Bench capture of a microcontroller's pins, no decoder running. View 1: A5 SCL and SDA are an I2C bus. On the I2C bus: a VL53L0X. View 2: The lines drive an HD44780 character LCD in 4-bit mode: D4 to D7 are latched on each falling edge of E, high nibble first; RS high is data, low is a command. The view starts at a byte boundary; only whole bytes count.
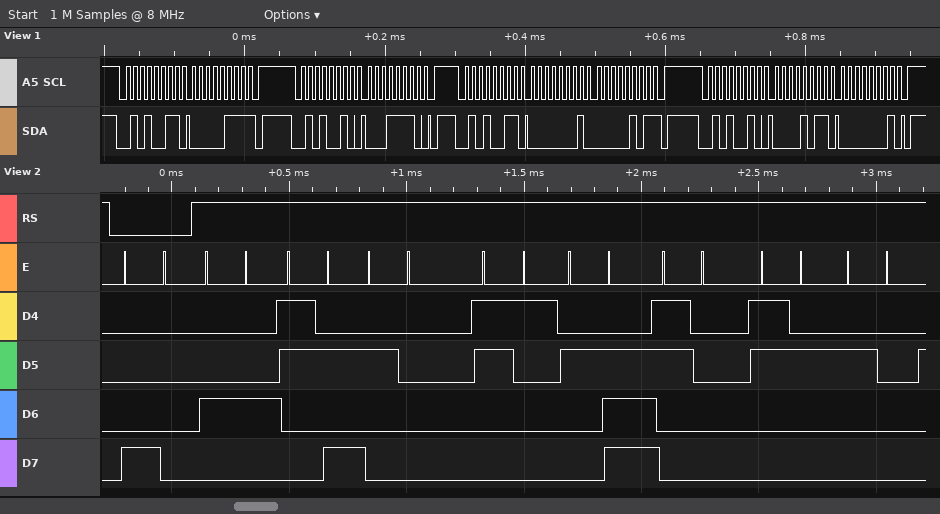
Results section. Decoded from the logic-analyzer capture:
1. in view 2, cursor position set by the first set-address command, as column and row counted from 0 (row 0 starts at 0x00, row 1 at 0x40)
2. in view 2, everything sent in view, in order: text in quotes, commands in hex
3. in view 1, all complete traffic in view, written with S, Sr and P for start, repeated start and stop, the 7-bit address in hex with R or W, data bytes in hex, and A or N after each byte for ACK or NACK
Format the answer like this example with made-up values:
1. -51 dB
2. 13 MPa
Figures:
1. column 0, row 0
2. 0x80 "D: 1.02 "
3. S 29R A 07 N P S 29W A 1E A P S 29R A 01 A 05 N P S 29W A 0B A 01 A P
